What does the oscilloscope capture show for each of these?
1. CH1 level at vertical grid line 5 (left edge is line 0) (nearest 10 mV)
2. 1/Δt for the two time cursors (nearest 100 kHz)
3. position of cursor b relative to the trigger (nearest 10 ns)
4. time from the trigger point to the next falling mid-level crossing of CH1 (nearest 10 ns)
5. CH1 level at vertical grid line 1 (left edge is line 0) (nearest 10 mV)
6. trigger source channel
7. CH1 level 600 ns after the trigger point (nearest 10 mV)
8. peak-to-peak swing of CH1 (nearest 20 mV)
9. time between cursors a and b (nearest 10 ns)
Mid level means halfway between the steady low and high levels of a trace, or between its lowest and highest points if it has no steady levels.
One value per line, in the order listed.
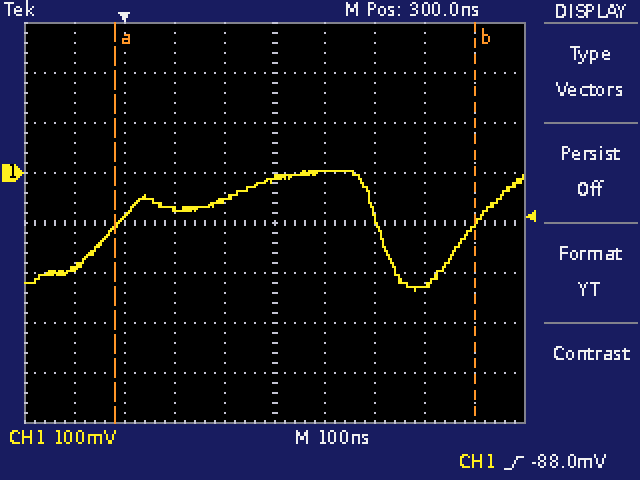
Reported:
-10 mV
1.4 MHz
+700 ns
510 ns
-190 mV
CH1
-220 mV
240 mV
720 ns
